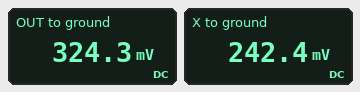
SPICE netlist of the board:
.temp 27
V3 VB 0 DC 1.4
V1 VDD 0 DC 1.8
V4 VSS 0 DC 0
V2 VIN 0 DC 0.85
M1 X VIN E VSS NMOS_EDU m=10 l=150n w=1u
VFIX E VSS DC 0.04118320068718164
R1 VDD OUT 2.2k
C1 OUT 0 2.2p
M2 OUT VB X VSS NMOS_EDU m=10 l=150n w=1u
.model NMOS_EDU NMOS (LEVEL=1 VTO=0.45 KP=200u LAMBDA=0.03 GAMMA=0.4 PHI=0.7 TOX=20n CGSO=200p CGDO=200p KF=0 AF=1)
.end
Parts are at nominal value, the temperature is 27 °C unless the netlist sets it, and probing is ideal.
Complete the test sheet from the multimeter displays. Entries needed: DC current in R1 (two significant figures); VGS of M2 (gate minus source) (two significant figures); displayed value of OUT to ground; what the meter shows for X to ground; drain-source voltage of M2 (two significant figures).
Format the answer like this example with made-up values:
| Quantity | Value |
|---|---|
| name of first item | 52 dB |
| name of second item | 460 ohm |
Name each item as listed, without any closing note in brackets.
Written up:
| Quantity | Value |
|---|---|
| DC current in R1 | 670 µA |
| VGS of M2 (gate minus source) | 1.2 V |
| displayed value of OUT to ground | 324.3 mV |
| what the meter shows for X to ground | 242.4 mV |
| drain-source voltage of M2 | 82 mV |
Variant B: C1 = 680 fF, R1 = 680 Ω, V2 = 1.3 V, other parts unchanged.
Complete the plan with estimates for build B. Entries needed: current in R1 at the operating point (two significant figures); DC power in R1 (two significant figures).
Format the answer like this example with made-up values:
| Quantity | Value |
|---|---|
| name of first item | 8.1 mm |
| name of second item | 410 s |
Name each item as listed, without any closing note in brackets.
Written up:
| Quantity | Value |
|---|---|
| current in R1 at the operating point | 1.9 mA |
| DC power in R1 | 2.4 mW |
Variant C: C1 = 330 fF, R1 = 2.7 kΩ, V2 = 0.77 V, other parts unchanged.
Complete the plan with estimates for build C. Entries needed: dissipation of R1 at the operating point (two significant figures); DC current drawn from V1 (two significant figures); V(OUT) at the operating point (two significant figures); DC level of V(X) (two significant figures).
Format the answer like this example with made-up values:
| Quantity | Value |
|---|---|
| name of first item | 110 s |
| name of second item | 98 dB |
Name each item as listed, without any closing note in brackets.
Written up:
| Quantity | Value |
|---|---|
| dissipation of R1 at the operating point | 640 µW |
| DC current drawn from V1 | 490 µA |
| V(OUT) at the operating point | 480 mV |
| DC level of V(X) | 400 mV |
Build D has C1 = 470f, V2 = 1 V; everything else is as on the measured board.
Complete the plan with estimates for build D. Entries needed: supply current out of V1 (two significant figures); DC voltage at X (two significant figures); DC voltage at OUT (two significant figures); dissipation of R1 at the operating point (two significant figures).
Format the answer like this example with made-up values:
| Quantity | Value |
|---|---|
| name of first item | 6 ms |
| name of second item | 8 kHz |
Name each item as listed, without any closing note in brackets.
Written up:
| Quantity | Value |
|---|---|
| supply current out of V1 | 710 µA |
| DC voltage at X | 160 mV |
| DC voltage at OUT | 240 mV |
| dissipation of R1 at the operating point | 1.1 mW |
